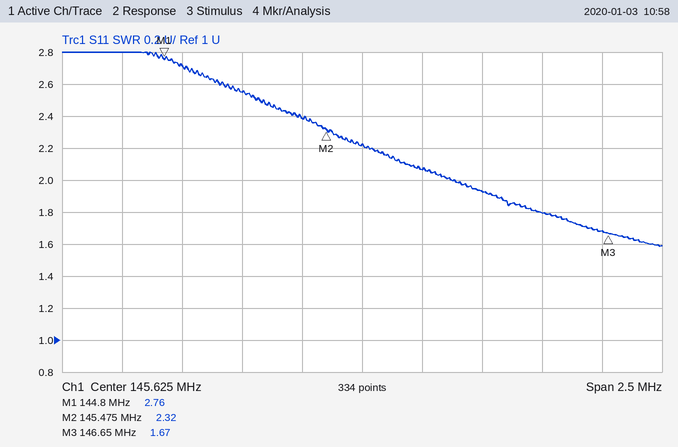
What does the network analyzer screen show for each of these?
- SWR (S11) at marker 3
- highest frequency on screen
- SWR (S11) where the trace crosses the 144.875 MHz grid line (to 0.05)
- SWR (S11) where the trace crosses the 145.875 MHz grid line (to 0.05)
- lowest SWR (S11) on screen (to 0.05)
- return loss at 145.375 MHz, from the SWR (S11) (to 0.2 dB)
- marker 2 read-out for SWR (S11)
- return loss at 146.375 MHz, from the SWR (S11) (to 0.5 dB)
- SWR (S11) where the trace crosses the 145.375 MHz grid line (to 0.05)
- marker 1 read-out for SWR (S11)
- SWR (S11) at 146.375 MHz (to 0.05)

1.67
146.875 MHz
2.70
2.05
1.60
7.8 dB
2.32
11.0 dB
2.40
2.76
1.80
